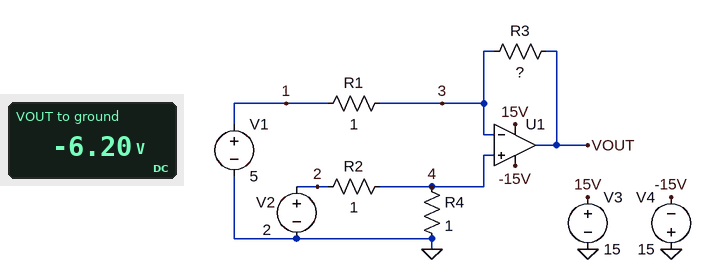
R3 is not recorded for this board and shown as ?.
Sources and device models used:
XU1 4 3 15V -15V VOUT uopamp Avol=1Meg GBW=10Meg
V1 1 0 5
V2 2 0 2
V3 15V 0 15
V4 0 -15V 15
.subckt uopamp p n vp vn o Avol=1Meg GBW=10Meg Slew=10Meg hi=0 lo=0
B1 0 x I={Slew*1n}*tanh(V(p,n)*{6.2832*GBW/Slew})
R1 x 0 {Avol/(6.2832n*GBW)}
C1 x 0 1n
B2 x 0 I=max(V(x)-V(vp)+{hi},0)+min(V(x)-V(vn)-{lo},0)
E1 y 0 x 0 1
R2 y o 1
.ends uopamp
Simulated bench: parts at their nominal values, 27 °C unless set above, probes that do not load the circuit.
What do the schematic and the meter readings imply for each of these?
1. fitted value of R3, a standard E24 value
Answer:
1.8 Ω
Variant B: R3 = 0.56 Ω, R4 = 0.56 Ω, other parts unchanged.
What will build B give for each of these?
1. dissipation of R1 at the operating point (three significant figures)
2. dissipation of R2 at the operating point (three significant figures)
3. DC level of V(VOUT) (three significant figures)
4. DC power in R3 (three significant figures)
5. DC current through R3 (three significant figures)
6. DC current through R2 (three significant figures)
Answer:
18.3 W
1.64 W
-1.68 V
10.3 W
4.28 A
1.28 A
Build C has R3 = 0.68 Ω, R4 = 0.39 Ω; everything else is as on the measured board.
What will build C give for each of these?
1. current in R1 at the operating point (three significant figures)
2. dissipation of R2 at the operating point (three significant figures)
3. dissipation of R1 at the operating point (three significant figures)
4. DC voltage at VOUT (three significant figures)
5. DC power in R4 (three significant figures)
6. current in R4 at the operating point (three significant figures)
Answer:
4.44 A
2.07 W
19.7 W
-2.46 V
807 mW
1.44 A
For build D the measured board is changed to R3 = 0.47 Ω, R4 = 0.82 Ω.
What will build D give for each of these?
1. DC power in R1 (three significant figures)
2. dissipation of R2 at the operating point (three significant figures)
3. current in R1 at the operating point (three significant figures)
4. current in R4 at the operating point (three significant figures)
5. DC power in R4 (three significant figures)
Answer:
16.8 W
1.21 W
4.10 A
1.10 A
990 mW
